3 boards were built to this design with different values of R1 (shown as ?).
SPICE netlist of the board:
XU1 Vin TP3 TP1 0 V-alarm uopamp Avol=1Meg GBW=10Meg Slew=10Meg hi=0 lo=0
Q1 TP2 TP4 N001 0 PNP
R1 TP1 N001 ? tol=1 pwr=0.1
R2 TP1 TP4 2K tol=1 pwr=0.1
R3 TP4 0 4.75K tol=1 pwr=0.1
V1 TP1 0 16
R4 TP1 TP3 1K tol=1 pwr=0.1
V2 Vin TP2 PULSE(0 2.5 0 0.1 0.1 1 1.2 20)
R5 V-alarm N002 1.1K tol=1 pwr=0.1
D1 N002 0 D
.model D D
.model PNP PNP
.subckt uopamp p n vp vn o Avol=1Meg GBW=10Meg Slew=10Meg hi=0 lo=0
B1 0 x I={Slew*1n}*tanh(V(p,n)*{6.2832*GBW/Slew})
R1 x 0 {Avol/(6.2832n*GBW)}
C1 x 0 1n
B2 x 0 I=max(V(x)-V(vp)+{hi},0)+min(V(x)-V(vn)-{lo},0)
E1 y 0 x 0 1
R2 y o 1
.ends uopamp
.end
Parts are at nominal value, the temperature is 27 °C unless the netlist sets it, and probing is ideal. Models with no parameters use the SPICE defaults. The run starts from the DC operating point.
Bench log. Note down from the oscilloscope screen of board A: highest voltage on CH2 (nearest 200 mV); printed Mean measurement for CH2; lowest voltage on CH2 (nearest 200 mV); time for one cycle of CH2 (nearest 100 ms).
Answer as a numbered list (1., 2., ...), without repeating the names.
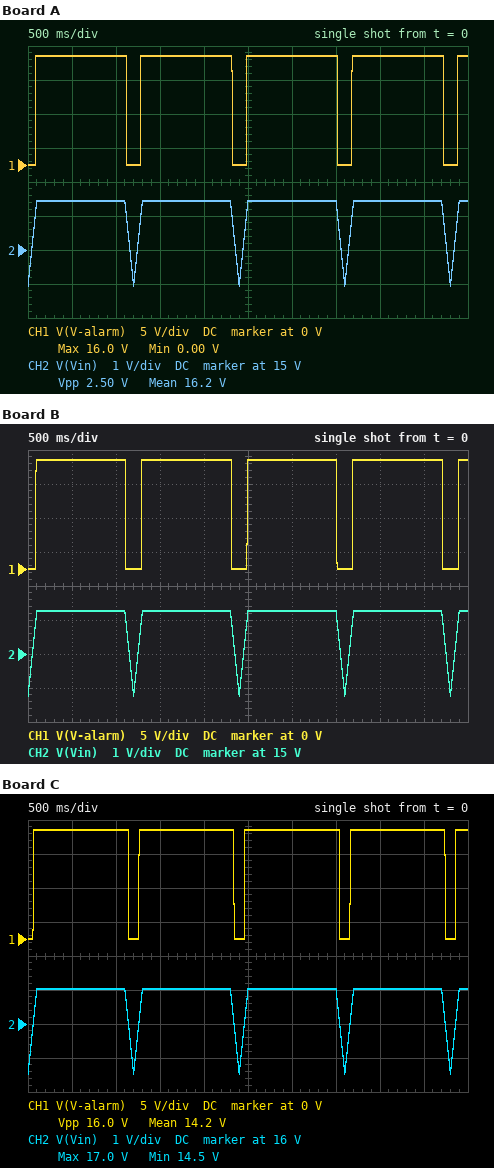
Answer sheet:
1. 16.4 V
2. 16.2 V
3. 14.0 V
4. 1.2 s
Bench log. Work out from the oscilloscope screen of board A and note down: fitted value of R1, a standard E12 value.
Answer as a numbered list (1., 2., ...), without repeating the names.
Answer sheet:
1. 1.5 kΩ
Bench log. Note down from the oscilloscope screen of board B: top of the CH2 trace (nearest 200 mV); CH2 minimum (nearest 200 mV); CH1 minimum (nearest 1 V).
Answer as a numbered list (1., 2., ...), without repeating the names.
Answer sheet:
1. 16.2 V
2. 13.8 V
3. 0 V
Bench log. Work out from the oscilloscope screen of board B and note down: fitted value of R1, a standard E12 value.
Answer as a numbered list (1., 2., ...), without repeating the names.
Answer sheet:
1. 1.8 kΩ
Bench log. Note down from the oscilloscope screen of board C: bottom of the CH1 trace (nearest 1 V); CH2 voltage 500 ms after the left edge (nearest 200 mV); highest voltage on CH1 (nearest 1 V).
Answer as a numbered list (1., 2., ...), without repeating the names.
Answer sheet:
1. 0 V
2. 17.0 V
3. 16 V
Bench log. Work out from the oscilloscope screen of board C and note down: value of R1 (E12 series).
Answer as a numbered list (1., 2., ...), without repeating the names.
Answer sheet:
1. 820 Ω
